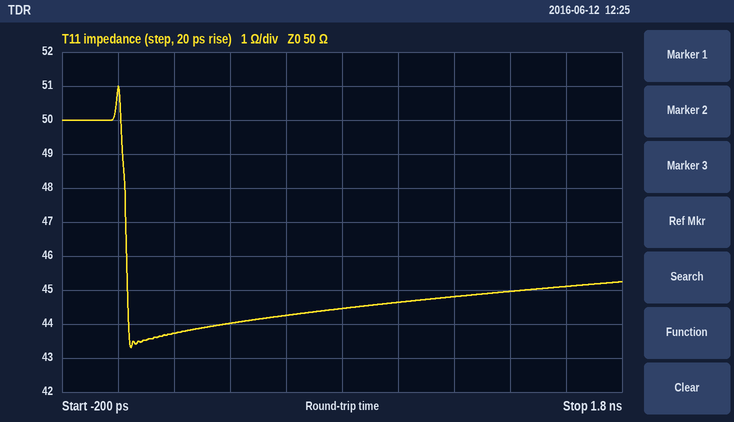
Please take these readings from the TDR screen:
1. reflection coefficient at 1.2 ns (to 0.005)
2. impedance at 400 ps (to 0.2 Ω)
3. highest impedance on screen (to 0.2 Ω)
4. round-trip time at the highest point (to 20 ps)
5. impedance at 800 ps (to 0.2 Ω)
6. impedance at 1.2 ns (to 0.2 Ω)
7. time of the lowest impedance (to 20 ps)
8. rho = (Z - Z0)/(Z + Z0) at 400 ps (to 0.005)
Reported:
-0.055
44.0 Ω
51.0 Ω
0 ps
44.4 Ω
44.8 Ω
40 ps
-0.065
